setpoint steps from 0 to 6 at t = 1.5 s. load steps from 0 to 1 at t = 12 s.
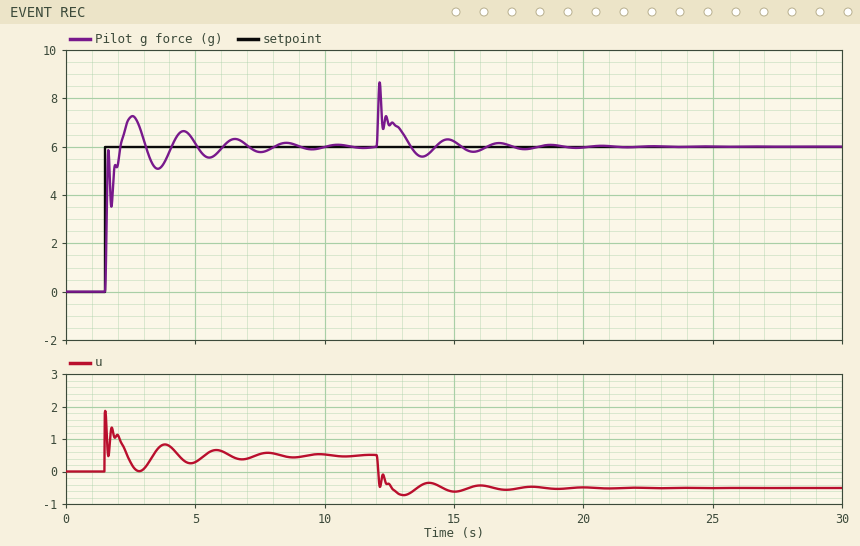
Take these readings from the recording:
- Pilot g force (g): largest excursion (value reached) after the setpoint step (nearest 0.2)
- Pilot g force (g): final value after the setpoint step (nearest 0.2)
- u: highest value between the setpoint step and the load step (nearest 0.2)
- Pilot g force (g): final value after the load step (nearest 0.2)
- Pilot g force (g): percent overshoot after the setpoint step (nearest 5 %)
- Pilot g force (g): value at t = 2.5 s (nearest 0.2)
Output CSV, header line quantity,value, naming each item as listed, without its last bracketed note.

quantity,value
Pilot g force (g): largest excursion (value reached) after the setpoint step,7.2
Pilot g force (g): final value after the setpoint step,6.0
u: highest value between the setpoint step and the load step,1.8
Pilot g force (g): final value after the load step,6.0
Pilot g force (g): percent overshoot after the setpoint step,20 %
Pilot g force (g): value at t = 2.5 s,7.2
